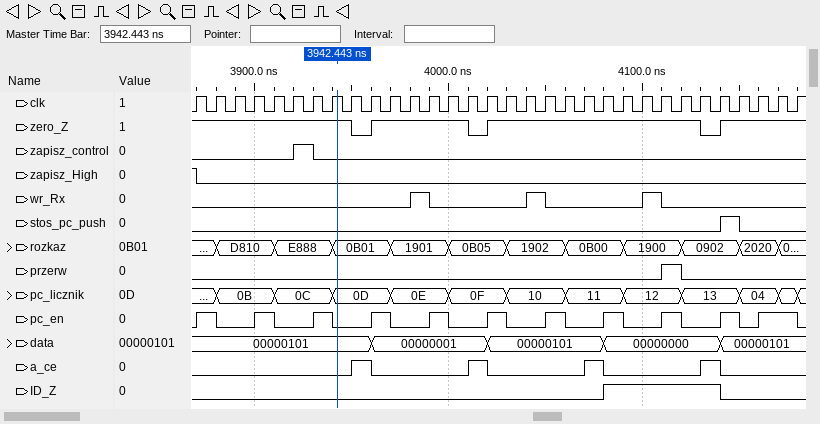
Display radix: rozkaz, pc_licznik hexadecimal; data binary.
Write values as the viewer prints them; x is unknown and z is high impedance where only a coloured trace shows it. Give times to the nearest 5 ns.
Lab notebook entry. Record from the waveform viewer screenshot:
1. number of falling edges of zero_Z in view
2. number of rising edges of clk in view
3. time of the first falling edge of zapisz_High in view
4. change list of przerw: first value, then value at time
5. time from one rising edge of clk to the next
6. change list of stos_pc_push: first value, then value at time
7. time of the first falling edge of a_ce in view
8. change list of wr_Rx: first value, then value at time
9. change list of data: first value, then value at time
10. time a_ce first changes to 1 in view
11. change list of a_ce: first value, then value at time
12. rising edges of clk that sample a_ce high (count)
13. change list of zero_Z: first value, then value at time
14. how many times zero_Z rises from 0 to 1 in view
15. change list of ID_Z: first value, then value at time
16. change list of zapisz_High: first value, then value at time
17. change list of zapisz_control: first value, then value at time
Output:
3
32
3870 ns
0, 1 at 4110 ns, 0 at 4120 ns
10 ns
0, 1 at 4140 ns, 0 at 4150 ns
3960 ns
0, 1 at 3980 ns, 0 at 3990 ns, 1 at 4040 ns, 0 at 4050 ns, 1 at 4100 ns, 0 at 4110 ns
00000101, 00000001 at 3960 ns, 00000101 at 4020 ns, 00000000 at 4080 ns, 00000101 at 4140 ns
3950 ns
0, 1 at 3950 ns, 0 at 3960 ns, 1 at 4010 ns, 0 at 4020 ns, 1 at 4070 ns, 0 at 4080 ns, 1 at 4130 ns, 0 at 4140 ns
4
1, 0 at 3950 ns, 1 at 3960 ns, 0 at 4010 ns, 1 at 4020 ns, 0 at 4130 ns, 1 at 4140 ns
3
0, 1 at 4080 ns, 0 at 4140 ns
1, 0 at 3870 ns
0, 1 at 3920 ns, 0 at 3930 ns
